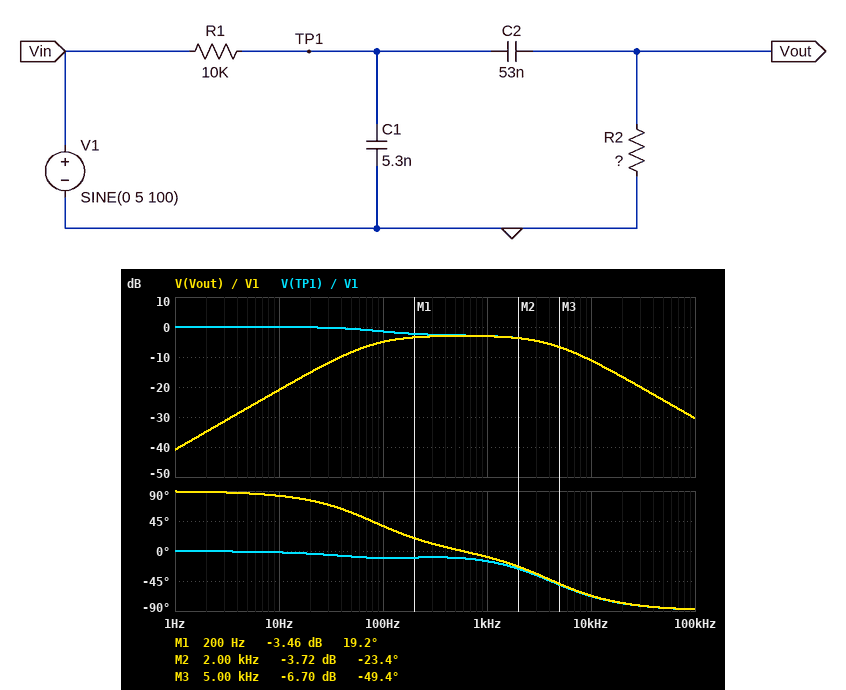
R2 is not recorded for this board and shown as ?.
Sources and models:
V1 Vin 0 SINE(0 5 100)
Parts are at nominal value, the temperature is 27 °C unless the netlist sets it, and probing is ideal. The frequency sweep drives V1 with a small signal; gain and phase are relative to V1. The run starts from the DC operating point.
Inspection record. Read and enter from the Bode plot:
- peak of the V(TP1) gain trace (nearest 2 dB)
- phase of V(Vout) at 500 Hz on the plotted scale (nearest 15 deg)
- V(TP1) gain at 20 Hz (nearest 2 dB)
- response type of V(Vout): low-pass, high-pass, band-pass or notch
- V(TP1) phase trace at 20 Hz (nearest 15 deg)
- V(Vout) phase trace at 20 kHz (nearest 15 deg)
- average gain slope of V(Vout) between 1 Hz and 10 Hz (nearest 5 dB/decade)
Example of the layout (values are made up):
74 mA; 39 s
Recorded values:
0 dB; 0 deg; 0 dB; band-pass; 0 deg; -75 deg; 20 dB/decade
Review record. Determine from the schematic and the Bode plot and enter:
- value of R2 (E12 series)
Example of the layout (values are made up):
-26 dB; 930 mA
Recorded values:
27 kΩ
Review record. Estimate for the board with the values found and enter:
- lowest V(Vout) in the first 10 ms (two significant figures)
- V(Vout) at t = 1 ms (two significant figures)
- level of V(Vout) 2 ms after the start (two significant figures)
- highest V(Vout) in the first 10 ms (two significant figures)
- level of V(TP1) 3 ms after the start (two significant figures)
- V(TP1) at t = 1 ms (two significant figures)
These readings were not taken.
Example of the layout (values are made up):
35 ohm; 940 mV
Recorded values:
-2.9 V; 1.6 V; 2.0 V; 2.0 V; 4.3 V; 2.2 V
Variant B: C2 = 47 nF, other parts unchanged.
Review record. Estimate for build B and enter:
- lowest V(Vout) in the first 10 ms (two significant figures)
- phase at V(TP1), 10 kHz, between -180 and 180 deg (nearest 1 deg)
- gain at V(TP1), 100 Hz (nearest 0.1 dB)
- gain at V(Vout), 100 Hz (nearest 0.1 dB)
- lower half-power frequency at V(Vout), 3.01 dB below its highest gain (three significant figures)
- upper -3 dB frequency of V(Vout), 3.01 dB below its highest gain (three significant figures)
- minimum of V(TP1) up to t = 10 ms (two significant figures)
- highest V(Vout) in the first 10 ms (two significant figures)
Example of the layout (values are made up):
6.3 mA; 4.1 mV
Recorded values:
-2.7 V; -68 deg; -1.3 dB; -5.4 dB; 87.0 Hz; 4.33 kHz; -4.3 V; 1.9 V
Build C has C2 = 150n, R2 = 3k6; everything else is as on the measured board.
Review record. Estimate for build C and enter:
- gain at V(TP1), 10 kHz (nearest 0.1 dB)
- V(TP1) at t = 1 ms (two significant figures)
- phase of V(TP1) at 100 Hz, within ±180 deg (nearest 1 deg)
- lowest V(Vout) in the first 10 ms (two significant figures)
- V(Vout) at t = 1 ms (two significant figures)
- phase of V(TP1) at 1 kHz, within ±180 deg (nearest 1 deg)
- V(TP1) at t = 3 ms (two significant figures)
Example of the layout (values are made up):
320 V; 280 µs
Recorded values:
-14.1 dB; 1.2 V; -34 deg; -1.1 V; 600 mV; -17 deg; 3.5 V
